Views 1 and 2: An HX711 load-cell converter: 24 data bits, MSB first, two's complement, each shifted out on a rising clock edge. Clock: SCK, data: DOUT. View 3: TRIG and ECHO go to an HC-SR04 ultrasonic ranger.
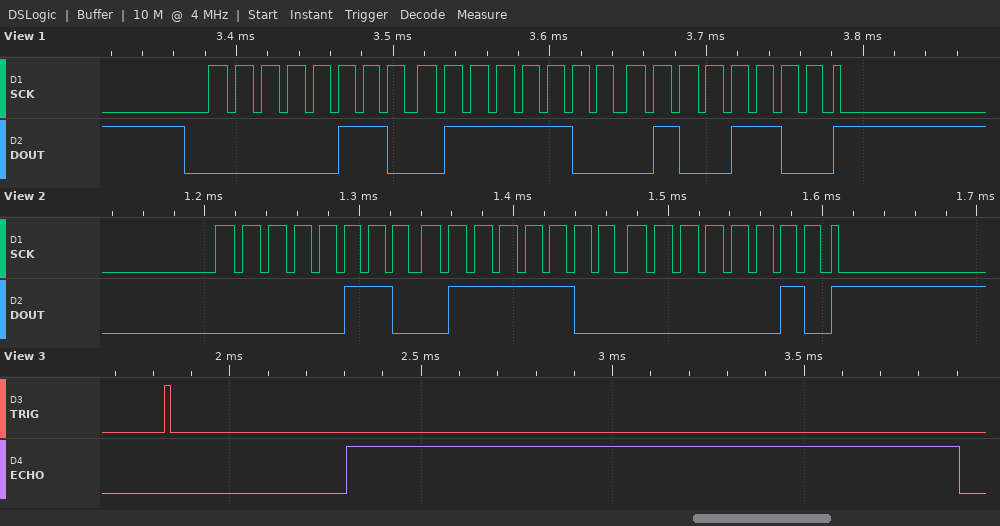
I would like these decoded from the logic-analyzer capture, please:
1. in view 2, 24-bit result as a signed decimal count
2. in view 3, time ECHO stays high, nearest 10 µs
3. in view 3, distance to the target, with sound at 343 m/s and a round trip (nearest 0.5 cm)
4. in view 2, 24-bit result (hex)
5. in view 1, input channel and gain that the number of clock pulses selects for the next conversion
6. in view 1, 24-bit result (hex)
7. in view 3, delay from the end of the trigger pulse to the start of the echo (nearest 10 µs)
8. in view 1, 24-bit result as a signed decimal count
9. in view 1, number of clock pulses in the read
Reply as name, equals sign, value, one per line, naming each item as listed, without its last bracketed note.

in view 2, 24-bit result as a signed decimal count = 424962
in view 3, time ECHO stays high, nearest 10 µs = 1600 µs
in view 3, distance to the target, with sound at 343 m/s and a round trip = 27.5 cm
in view 2, 24-bit result = 0x067C02
in view 1, input channel and gain that the number of clock pulses selects for the next conversion = channel A, gain 128
in view 1, 24-bit result = 0x067C4C
in view 3, delay from the end of the trigger pulse to the start of the echo = 460 µs
in view 1, 24-bit result as a signed decimal count = 425036
in view 1, number of clock pulses in the read = 25
